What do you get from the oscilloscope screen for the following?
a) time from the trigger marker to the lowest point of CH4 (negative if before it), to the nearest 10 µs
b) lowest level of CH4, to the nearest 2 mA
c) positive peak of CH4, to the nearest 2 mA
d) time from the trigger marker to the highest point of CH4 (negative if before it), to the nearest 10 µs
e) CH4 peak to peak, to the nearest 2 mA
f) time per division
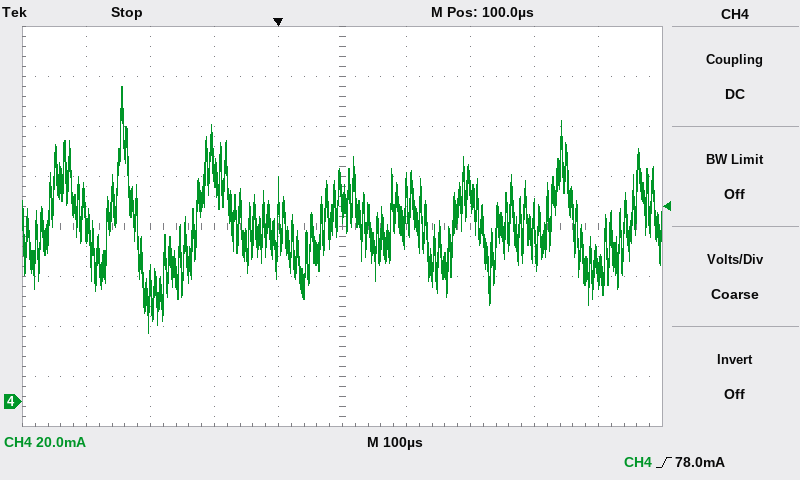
-200 µs
28 mA
126 mA
-240 µs
98 mA
100 µs
